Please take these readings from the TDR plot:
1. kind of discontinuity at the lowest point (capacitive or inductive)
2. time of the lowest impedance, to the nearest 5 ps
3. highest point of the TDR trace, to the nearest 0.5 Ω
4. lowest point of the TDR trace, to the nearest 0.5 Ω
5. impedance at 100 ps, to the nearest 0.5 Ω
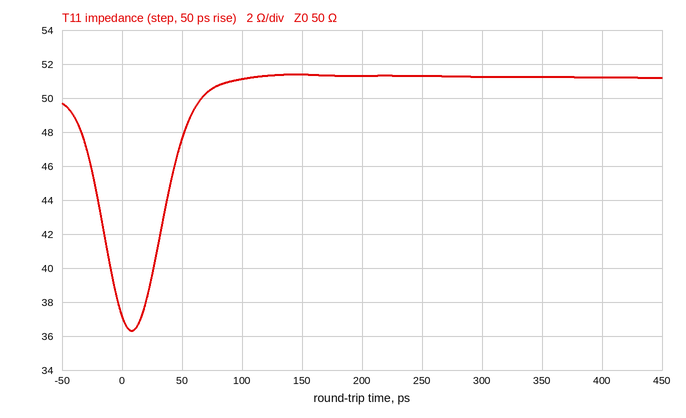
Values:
capacitive
10 ps
51.5 Ω
36.5 Ω
51.0 Ω
